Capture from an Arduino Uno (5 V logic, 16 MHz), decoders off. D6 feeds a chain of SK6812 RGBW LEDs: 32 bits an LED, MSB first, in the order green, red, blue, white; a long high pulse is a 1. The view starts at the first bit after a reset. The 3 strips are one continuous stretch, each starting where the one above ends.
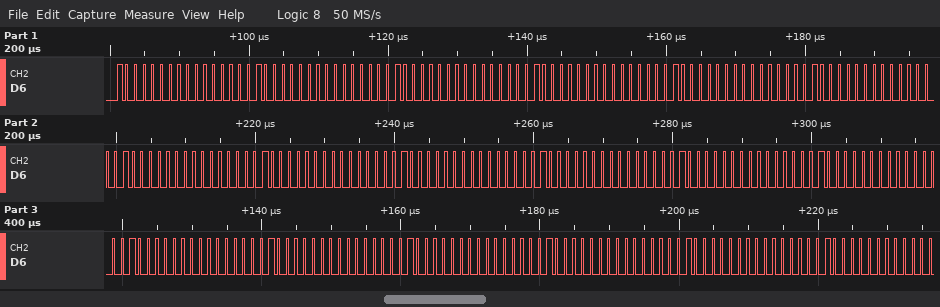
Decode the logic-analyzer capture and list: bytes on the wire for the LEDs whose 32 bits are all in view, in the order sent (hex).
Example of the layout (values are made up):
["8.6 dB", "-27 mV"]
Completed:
["80 00 80 00 80 00 80 00 80 00 80 00 80 00 80 00 80 00 80 00 80 00 80 00 80 00 80 00 80 00 80 00"]
